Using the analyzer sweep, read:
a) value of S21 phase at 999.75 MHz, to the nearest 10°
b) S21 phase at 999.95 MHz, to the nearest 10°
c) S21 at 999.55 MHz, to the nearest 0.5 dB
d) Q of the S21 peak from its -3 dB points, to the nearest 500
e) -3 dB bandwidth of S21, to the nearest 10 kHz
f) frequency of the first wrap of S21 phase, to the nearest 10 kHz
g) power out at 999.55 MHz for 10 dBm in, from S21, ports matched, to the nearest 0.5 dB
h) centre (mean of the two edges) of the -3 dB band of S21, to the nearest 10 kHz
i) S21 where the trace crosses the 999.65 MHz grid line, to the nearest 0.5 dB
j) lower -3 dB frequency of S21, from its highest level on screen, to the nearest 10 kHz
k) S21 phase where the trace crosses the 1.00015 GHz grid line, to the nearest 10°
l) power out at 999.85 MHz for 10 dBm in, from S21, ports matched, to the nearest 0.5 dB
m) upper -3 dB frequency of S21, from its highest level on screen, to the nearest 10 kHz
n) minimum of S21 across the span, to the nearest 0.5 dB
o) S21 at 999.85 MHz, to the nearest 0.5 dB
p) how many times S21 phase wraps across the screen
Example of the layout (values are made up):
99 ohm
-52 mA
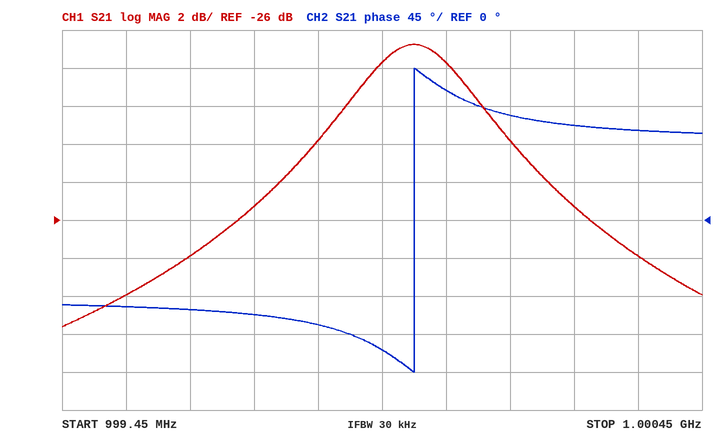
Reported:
-110°
-150°
-30.0 dB
5000
200 kHz
1.00000 GHz
-20.0 dBm
1.00000 GHz
-28.0 dB
999.90 MHz
120°
-12.0 dBm
1.00010 GHz
-31.5 dB
-22.0 dB
1
